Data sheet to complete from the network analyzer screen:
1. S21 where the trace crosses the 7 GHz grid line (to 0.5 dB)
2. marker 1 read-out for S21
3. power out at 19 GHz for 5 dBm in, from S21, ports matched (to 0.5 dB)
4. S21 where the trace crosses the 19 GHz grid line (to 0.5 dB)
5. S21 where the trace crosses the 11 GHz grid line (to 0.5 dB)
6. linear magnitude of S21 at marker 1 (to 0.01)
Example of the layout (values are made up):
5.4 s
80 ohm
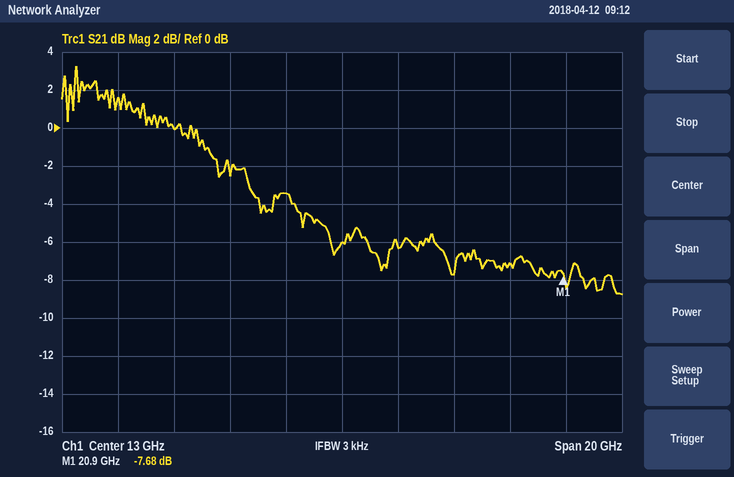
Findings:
0.0 dB
-7.68 dB
-2.0 dBm
-7.0 dB
-3.5 dB
0.41
